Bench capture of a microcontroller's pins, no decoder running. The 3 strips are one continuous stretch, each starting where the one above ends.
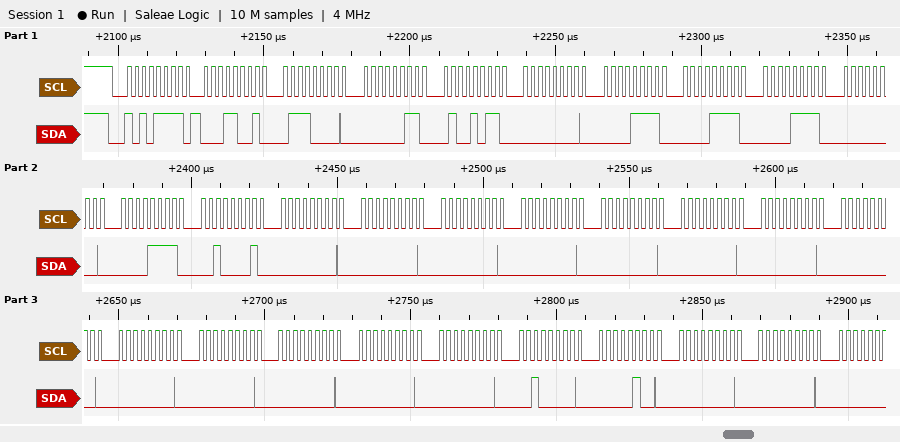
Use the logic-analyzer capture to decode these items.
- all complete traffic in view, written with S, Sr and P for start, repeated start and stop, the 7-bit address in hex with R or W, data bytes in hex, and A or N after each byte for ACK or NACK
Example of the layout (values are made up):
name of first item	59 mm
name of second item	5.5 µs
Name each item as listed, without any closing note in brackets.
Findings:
all complete traffic in view, written with S, Sr and P for start, repeated start and stop, the 7-bit address in hex with R or W, data bytes in hex, and A or N after each byte for ACK or NACK	S 57R A 19 A 70 A 03 A 4B A 00 A 0F A 0F A 0F A 00 A 0F A 21 A 00 A 00 A 00 A 00 A 00 A 00 A 00 A 00 A 00 A 00 A 00 A 00 A 00 A 20 A 04 A 00 A 00 A
